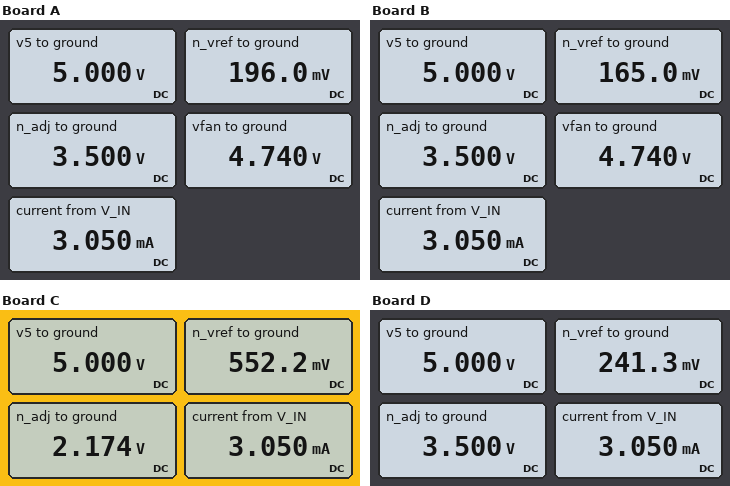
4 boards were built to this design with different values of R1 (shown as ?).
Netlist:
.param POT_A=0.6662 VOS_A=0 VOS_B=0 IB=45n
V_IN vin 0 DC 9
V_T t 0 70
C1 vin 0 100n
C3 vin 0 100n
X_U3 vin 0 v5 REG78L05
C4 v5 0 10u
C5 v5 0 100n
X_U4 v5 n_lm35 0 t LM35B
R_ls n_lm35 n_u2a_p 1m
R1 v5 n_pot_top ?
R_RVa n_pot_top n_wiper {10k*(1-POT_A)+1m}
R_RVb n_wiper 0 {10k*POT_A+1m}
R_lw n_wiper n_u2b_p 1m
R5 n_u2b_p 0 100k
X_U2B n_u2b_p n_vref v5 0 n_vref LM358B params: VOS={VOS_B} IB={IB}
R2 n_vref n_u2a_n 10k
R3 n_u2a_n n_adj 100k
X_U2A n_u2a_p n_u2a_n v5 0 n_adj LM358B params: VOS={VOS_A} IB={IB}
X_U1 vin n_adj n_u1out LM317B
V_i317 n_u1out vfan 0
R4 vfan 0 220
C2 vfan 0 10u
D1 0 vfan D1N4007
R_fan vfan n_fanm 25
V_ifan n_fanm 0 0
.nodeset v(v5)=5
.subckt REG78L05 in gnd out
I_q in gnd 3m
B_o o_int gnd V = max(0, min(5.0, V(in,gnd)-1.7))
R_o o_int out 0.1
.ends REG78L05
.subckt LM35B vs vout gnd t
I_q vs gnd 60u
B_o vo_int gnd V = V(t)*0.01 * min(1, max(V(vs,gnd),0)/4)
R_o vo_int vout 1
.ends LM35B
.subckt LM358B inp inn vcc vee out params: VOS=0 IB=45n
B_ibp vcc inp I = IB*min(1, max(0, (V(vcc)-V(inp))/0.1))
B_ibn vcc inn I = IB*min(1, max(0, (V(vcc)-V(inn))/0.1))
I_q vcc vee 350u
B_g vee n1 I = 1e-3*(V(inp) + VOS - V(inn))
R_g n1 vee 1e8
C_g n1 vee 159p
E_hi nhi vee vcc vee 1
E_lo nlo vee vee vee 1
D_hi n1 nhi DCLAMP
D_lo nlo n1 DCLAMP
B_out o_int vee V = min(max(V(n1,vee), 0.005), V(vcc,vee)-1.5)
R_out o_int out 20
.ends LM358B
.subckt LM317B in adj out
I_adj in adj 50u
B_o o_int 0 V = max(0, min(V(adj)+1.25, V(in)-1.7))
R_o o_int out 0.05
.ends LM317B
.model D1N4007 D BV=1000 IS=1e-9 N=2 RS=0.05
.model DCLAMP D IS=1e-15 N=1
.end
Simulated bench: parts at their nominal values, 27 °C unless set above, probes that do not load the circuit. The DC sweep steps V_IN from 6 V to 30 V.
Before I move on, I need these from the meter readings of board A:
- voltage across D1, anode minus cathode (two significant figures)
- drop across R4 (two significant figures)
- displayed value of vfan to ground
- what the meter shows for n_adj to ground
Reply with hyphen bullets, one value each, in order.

- -4.7 V
- 4.7 V
- 4.740 V
- 3.500 V
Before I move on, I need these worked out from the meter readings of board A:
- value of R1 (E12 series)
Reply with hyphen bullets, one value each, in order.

- 150 kΩ
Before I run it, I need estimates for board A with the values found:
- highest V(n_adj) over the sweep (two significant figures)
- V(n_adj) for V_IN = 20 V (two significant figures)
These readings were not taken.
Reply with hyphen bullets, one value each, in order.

- 3.5 V
- 3.5 V
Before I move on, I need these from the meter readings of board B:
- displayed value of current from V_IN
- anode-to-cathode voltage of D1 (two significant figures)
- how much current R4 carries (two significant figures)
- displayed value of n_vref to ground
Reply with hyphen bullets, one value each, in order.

- 3.050 mA
- -4.7 V
- 22 mA
- 165.0 mV
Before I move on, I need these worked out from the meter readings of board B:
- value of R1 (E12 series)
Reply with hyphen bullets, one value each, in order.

- 180 kΩ
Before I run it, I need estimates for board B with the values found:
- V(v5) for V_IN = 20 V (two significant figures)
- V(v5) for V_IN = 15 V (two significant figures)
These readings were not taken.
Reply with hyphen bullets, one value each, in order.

- 5.0 V
- 5.0 V
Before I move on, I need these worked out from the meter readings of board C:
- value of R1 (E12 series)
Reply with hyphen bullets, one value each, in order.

- 47 kΩ
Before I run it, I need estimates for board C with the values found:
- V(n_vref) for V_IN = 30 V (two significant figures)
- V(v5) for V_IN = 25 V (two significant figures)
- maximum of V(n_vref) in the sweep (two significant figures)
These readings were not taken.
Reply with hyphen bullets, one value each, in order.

- 550 mV
- 5.0 V
- 550 mV
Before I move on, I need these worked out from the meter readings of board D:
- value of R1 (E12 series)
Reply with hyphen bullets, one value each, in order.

- 120 kΩ
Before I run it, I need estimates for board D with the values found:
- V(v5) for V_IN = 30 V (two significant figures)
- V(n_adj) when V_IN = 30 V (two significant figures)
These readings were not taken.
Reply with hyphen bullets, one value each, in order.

- 5.0 V
- 3.5 V
